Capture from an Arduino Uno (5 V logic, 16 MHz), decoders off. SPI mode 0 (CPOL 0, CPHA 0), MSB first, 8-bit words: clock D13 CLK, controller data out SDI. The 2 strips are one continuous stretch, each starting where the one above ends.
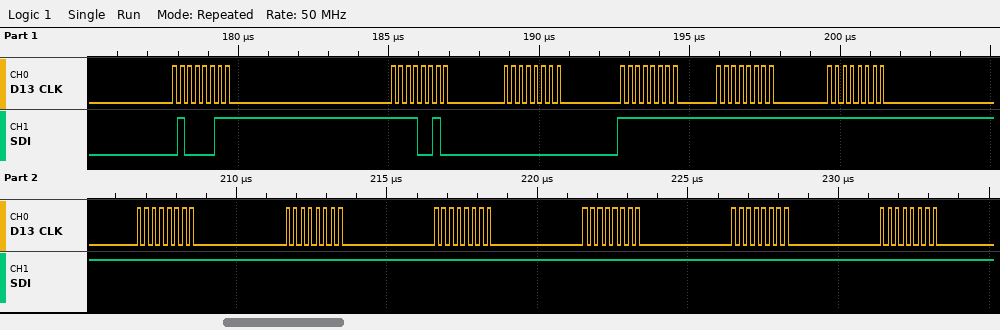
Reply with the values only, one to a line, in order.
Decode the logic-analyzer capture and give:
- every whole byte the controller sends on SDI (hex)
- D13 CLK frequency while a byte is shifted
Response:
0x43 0xF2 0x00 0xFF 0xFF 0xFF 0xFF 0xFF 0xFF 0xFF 0xFF 0xFF
4 MHz
